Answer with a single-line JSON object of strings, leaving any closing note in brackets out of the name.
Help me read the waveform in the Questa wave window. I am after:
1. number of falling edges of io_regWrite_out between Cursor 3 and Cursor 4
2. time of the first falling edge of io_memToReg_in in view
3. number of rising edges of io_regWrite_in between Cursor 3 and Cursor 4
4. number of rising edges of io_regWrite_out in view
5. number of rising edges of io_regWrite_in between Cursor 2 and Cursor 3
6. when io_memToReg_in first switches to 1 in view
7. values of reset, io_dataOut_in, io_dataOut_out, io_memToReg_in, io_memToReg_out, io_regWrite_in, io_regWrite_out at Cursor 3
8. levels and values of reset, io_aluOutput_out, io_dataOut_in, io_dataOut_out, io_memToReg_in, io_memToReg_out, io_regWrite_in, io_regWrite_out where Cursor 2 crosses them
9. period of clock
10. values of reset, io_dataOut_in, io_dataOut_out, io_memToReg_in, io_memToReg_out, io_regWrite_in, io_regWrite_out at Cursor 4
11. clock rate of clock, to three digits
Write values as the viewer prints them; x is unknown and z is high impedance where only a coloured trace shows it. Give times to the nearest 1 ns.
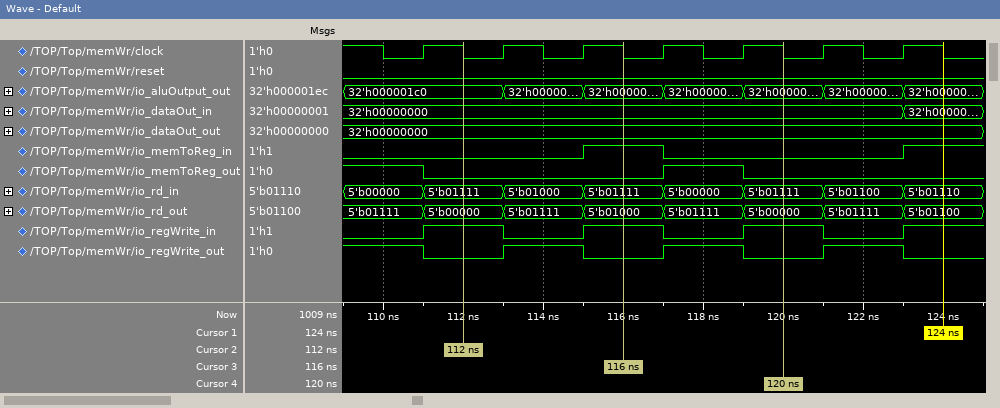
{"number of falling edges of io_regWrite_out between Cursor 3 and Cursor 4": "1", "time of the first falling edge of io_memToReg_in in view": "117 ns", "number of rising edges of io_regWrite_in between Cursor 3 and Cursor 4": "1", "number of rising edges of io_regWrite_out in view": "3", "number of rising edges of io_regWrite_in between Cursor 2 and Cursor 3": "1", "when io_memToReg_in first switches to 1 in view": "115 ns", "values of reset, io_dataOut_in, io_dataOut_out, io_memToReg_in, io_memToReg_out, io_regWrite_in, io_regWrite_out at Cursor 3": "reset=0, io_dataOut_in=32'h00000000, io_dataOut_out=32'h00000000, io_memToReg_in=1, io_memToReg_out=0, io_regWrite_in=1, io_regWrite_out=0", "levels and values of reset, io_aluOutput_out, io_dataOut_in, io_dataOut_out, io_memToReg_in, io_memToReg_out, io_regWrite_in, io_regWrite_out where Cursor 2 crosses them": "reset=0, io_aluOutput_out=32'h000001c0, io_dataOut_in=32'h00000000, io_dataOut_out=32'h00000000, io_memToReg_in=0, io_memToReg_out=0, io_regWrite_in=1, io_regWrite_out=0", "period of clock": "2 ns", "values of reset, io_dataOut_in, io_dataOut_out, io_memToReg_in, io_memToReg_out, io_regWrite_in, io_regWrite_out at Cursor 4": "reset=0, io_dataOut_in=32'h00000000, io_dataOut_out=32'h00000000, io_memToReg_in=0, io_memToReg_out=0, io_regWrite_in=1, io_regWrite_out=0", "clock rate of clock, to three digits": "500 MHz"}
